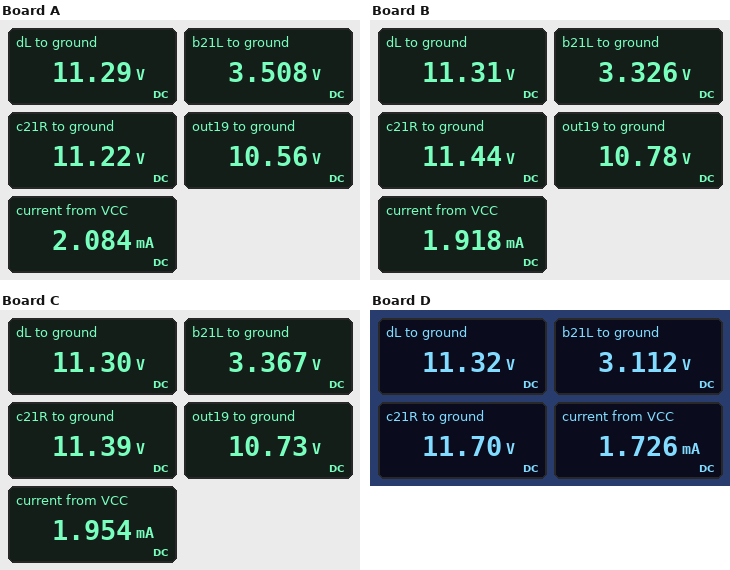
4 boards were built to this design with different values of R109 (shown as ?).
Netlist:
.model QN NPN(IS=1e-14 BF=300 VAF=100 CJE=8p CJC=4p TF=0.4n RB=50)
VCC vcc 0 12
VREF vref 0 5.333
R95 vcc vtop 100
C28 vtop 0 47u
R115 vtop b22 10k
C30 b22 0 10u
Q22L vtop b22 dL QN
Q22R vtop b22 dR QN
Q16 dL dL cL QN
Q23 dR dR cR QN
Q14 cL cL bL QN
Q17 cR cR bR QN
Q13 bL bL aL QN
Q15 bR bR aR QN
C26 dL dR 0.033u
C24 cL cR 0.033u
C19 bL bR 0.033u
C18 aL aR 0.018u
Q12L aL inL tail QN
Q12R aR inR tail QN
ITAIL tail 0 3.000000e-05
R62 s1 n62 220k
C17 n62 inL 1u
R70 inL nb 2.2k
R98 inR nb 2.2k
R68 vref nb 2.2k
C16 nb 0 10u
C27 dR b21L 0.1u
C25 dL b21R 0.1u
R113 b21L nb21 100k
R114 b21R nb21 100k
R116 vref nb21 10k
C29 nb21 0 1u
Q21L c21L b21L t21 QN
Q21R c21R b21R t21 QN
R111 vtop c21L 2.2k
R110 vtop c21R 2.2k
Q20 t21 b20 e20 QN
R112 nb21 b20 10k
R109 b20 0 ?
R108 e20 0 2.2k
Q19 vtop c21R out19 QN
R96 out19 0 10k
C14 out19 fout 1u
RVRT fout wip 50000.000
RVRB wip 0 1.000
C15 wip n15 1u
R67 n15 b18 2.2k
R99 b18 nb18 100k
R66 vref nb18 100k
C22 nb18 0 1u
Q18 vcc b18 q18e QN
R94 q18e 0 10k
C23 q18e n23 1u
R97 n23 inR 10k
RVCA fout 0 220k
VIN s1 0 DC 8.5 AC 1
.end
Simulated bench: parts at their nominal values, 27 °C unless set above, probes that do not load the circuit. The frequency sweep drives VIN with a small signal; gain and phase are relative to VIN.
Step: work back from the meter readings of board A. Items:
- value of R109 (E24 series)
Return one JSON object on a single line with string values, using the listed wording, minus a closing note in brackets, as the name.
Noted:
{"value of R109": "11 kΩ"}
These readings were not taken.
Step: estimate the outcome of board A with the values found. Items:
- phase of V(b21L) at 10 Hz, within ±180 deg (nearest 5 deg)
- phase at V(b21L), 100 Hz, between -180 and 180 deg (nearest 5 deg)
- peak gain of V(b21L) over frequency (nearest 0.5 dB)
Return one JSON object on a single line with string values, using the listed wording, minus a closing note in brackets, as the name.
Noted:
{"phase of V(b21L) at 10 Hz, within ±180 deg": "85 deg", "phase at V(b21L), 100 Hz, between -180 and 180 deg": "0 deg", "peak gain of V(b21L) over frequency": "-49.0 dB"}
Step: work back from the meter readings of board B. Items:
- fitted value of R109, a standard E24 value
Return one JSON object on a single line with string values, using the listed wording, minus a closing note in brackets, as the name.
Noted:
{"fitted value of R109, a standard E24 value": "7.5 kΩ"}
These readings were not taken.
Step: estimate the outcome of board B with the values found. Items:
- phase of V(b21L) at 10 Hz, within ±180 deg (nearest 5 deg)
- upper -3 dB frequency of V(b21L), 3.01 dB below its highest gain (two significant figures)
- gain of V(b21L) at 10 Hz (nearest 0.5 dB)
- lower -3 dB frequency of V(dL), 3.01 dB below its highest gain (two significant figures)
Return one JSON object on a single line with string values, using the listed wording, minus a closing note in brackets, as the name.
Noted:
{"phase of V(b21L) at 10 Hz, within ±180 deg": "80 deg", "upper -3 dB frequency of V(b21L), 3.01 dB below its highest gain": "290 Hz", "gain of V(b21L) at 10 Hz": "-60.0 dB", "lower -3 dB frequency of V(dL), 3.01 dB below its highest gain": "810 mHz"}
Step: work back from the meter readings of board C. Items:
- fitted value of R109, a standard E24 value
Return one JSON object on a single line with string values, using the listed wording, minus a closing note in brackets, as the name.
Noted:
{"fitted value of R109, a standard E24 value": "8.2 kΩ"}
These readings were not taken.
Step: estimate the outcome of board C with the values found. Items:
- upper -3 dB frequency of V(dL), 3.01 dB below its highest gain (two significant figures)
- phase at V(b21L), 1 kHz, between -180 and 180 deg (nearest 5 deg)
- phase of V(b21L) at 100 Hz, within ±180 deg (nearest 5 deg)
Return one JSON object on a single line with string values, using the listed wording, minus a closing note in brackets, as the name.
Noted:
{"upper -3 dB frequency of V(dL), 3.01 dB below its highest gain": "160 Hz", "phase at V(b21L), 1 kHz, between -180 and 180 deg": "-130 deg", "phase of V(b21L) at 100 Hz, within ±180 deg": "-5 deg"}
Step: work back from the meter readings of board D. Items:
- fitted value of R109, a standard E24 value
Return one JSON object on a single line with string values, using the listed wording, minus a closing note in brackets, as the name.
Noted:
{"fitted value of R109, a standard E24 value": "4.3 kΩ"}
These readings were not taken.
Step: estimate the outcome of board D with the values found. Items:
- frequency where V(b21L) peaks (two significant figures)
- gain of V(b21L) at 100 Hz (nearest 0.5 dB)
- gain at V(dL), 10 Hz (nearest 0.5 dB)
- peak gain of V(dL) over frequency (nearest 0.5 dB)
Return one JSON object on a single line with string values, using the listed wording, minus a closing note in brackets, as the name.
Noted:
{"frequency where V(b21L) peaks": "76 Hz", "gain of V(b21L) at 100 Hz": "-47.5 dB", "gain at V(dL), 10 Hz": "-45.5 dB", "peak gain of V(dL) over frequency": "-45.5 dB"}
